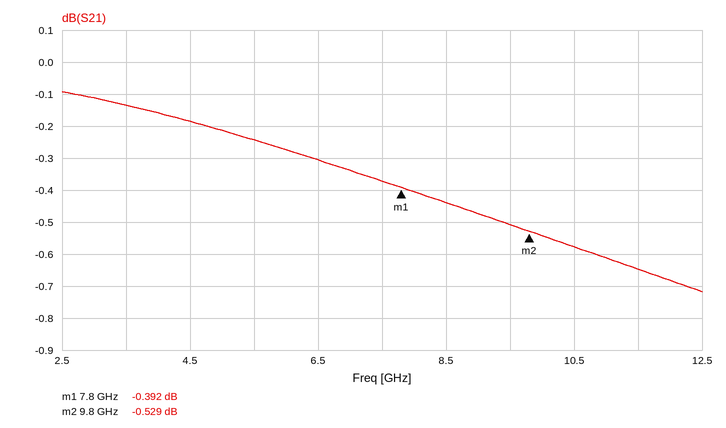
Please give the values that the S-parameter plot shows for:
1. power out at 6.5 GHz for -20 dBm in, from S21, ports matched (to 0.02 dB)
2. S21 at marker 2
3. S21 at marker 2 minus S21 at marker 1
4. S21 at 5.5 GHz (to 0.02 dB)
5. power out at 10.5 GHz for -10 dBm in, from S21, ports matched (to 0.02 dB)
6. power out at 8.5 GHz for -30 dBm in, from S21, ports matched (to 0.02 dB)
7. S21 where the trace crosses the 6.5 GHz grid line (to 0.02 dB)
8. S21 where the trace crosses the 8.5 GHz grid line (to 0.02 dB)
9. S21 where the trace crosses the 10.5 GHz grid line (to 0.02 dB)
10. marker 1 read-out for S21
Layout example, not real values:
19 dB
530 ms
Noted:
-20.30 dBm
-0.529 dB
-0.137 dB
-0.24 dB
-10.58 dBm
-30.44 dBm
-0.30 dB
-0.44 dB
-0.58 dB
-0.392 dB
